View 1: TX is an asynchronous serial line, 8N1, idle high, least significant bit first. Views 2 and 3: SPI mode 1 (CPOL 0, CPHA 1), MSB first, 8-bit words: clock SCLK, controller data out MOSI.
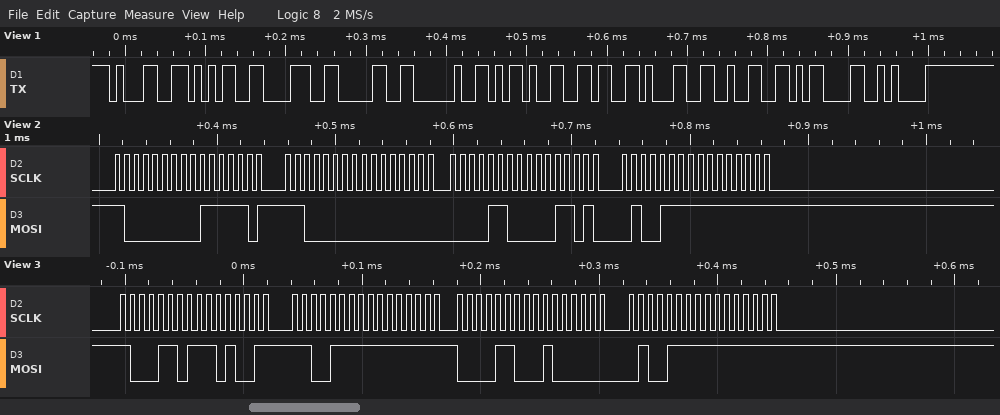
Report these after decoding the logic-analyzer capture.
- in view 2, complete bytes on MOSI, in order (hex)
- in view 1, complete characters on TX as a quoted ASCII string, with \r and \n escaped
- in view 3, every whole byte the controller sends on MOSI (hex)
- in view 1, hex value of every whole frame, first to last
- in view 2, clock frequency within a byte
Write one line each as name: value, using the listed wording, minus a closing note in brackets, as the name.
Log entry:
in view 2, complete bytes on MOSI, in order: 80 7D C0 00 0C 1A 4F FF
in view 1, complete characters on TX as a quoted ASCII string, with \r and \n escaped: "1580 -612\r\n"
in view 3, every whole byte the controller sends on MOSI: 8D D3 CF FF 0C 40 4F FF
in view 1, hex value of every whole frame, first to last: 0x31 0x35 0x38 0x30 0x20 0x2D 0x36 0x31 0x32 0x0D 0x0A
in view 2, clock frequency within a byte: 125 kHz
